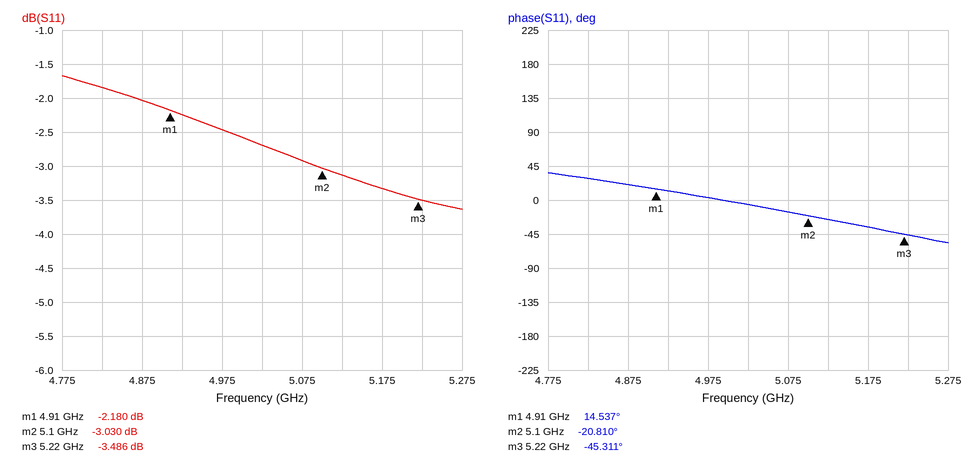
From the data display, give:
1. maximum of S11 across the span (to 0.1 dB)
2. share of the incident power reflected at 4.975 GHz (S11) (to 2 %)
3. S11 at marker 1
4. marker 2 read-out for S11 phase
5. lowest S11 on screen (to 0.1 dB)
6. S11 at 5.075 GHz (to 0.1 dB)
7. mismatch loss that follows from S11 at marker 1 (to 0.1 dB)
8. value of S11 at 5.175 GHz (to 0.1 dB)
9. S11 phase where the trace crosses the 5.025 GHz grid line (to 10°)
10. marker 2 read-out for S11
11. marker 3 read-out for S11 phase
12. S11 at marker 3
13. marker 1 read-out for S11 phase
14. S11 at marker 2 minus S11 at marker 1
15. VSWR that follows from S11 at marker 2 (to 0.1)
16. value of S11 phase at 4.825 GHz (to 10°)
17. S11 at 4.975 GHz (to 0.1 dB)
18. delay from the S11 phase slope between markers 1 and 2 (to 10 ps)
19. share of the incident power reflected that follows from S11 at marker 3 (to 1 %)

-1.7 dB
56 %
-2.180 dB
-20.810°
-3.6 dB
-2.9 dB
4.0 dB
-3.3 dB
-10°
-3.030 dB
-45.311°
-3.486 dB
14.537°
-0.850 dB
5.8
30°
-2.5 dB
520 ps
45 %
